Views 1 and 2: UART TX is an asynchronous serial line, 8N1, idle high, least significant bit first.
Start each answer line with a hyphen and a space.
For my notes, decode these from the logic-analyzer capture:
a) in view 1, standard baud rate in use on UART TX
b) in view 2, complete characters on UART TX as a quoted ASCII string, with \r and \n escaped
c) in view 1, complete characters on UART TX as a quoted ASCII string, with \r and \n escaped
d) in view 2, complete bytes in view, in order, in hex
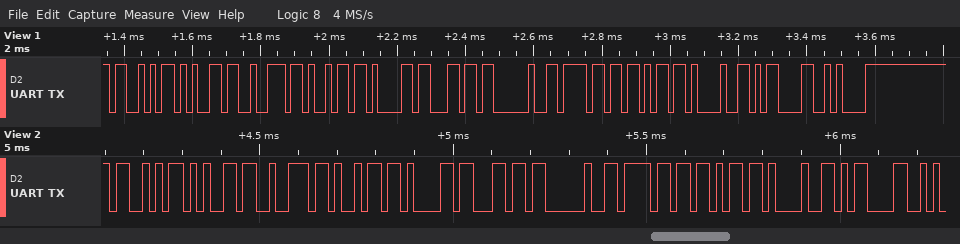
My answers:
- 57600 baud
- "Serial ok!\r"
- "Serial ok!\r\n"
- 53 65 72 69 61 6C 20 6F 6B 21 0D
